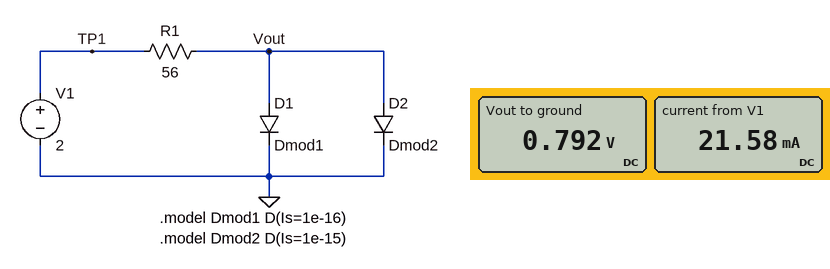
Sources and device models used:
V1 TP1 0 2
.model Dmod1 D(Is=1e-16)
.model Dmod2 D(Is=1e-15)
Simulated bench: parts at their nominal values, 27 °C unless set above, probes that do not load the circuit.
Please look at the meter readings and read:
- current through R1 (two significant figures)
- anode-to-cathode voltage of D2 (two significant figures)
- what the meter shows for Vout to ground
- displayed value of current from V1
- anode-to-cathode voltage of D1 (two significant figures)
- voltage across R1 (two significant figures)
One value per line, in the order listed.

22 mA
790 mV
0.792 V
21.58 mA
790 mV
1.2 V
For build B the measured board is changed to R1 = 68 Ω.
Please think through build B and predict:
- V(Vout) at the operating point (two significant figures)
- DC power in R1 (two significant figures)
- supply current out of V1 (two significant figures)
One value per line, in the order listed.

790 mV
22 mW
18 mA
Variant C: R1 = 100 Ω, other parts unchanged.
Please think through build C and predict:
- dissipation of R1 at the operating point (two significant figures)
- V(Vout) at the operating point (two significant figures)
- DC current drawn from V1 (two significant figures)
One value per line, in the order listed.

15 mW
780 mV
12 mA
